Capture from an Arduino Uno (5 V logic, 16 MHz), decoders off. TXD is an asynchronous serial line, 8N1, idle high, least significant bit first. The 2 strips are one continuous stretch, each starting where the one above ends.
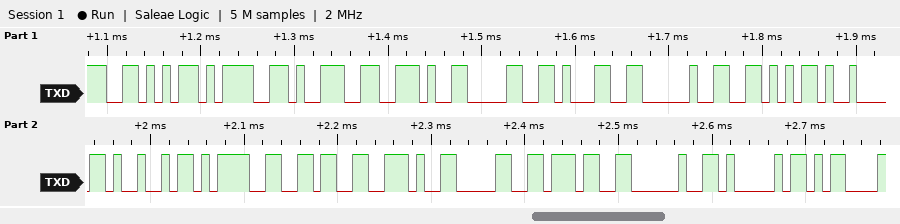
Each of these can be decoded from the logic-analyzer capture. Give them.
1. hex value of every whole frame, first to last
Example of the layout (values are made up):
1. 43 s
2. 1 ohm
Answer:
1. 56 3D 39 2E 30 31 20 56 09 49 3D 36 2E 30 37 20 41 0D
